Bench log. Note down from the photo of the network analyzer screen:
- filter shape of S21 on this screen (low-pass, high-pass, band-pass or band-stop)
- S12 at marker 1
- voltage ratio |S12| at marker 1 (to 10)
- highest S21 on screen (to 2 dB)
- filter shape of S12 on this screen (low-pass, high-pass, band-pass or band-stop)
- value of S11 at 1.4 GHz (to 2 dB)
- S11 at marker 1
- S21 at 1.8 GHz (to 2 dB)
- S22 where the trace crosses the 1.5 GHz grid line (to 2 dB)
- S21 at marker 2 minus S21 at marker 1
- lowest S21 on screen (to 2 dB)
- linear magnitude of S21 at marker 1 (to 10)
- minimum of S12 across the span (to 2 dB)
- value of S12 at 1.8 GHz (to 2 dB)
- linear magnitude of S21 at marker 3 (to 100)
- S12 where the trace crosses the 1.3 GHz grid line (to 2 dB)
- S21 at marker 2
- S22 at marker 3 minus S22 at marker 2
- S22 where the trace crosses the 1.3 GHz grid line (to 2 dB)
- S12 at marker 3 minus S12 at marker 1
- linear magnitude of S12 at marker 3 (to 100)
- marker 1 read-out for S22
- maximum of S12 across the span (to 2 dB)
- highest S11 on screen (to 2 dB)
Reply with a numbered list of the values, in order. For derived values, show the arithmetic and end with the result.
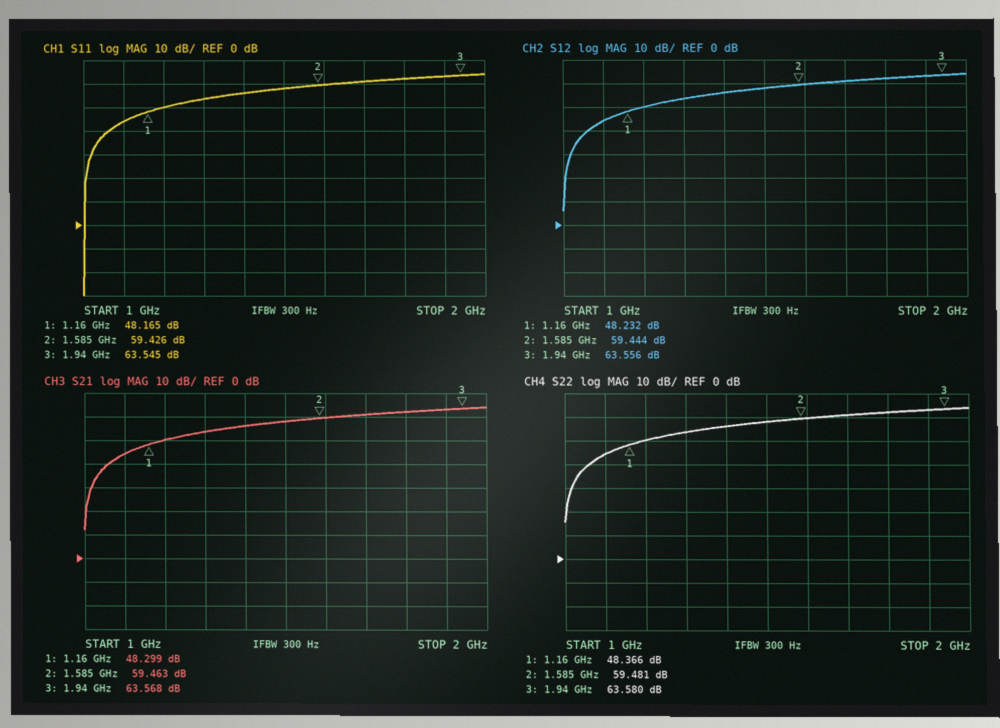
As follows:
1. high-pass
2. 48.232 dB
3. 10^(48.232/20) ≈ 258, so 260 to the nearest 10
4. 64 dB
5. high-pass
6. 56 dB
7. 48.165 dB
8. 62 dB
9. 58 dB
10. 59.463 − (48.299) = 11.164 dB
11. 12 dB
12. 10^(48.299/20) ≈ 260
13. 6 dB
14. 62 dB
15. 10^(63.568/20) ≈ 1508, so 1500 to the nearest 100
16. 54 dB
17. 59.463 dB
18. 63.58 − (59.481) = 4.099 dB
19. 54 dB
20. 63.556 − (48.232) = 15.324 dB
21. 10^(63.556/20) ≈ 1506, so 1500 to the nearest 100
22. 48.366 dB
23. 64 dB
24. 64 dB
